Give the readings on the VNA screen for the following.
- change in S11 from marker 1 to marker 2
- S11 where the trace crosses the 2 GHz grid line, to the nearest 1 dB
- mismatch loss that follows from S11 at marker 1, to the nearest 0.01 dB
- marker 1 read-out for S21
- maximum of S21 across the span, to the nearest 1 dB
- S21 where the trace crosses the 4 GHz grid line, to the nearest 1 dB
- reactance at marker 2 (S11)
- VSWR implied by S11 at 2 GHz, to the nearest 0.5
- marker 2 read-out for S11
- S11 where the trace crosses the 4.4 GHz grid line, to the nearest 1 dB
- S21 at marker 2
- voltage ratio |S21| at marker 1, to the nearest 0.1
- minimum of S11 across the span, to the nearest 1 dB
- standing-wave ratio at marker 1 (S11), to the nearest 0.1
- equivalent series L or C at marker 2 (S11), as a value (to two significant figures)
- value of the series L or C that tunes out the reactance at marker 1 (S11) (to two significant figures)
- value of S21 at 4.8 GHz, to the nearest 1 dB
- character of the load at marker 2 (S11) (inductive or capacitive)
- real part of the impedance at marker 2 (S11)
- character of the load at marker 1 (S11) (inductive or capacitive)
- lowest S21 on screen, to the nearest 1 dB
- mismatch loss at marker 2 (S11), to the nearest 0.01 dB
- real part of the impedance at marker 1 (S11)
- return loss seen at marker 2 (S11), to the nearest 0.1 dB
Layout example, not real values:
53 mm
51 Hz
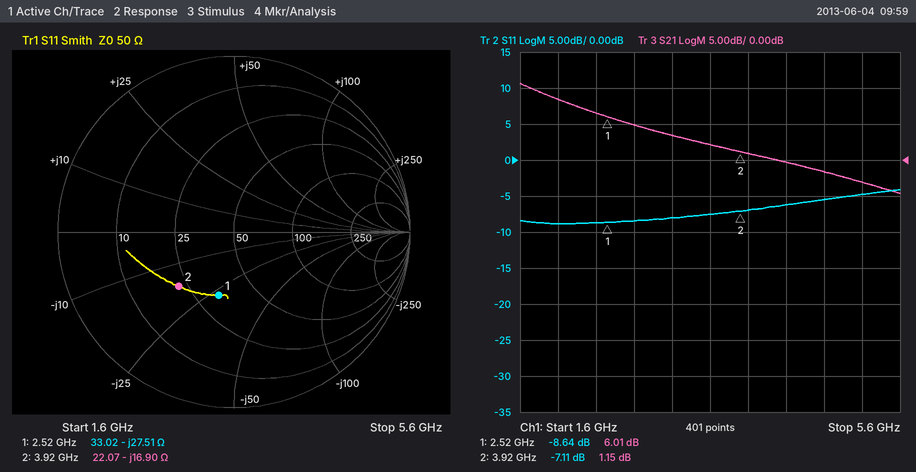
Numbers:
1.53 dB
-9 dB
0.64 dB
6.01 dB
11 dB
1 dB
-16.90 Ω
2.0
-7.11 dB
-6 dB
1.15 dB
2.0
-9 dB
2.2
2.4 pF
1.7 nH
-2 dB
capacitive
22.07 Ω
capacitive
-5 dB
0.94 dB
33.02 Ω
7.1 dB
